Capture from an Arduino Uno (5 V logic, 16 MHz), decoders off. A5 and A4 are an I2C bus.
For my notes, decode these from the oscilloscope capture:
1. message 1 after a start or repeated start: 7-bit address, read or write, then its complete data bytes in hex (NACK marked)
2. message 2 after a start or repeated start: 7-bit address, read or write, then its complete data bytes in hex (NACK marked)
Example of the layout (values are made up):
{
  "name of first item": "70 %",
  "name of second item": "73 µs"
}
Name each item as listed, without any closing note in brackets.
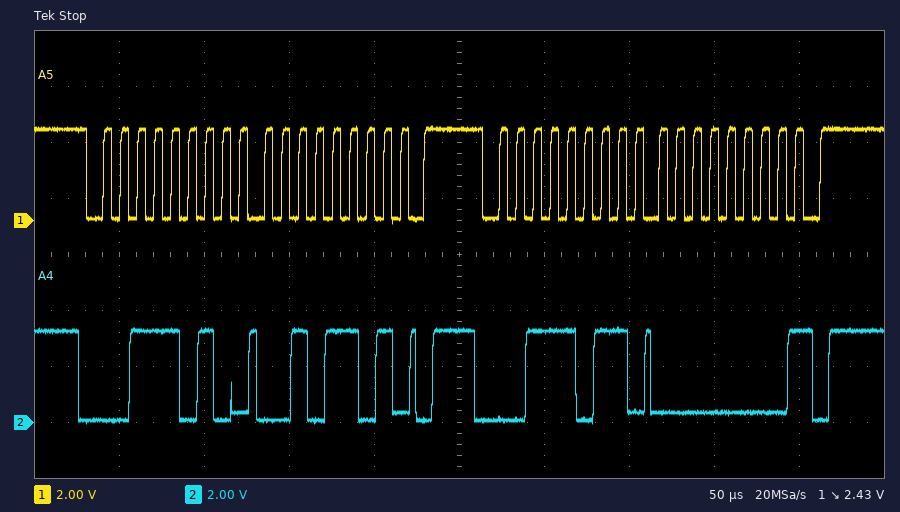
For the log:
{
  "message 1 after a start or repeated start: 7-bit address, read or write, then its complete data bytes in hex": "0x1D write: 2D",
  "message 2 after a start or repeated start: 7-bit address, read or write, then its complete data bytes in hex": "0x1D read: 00 NACK"
}
